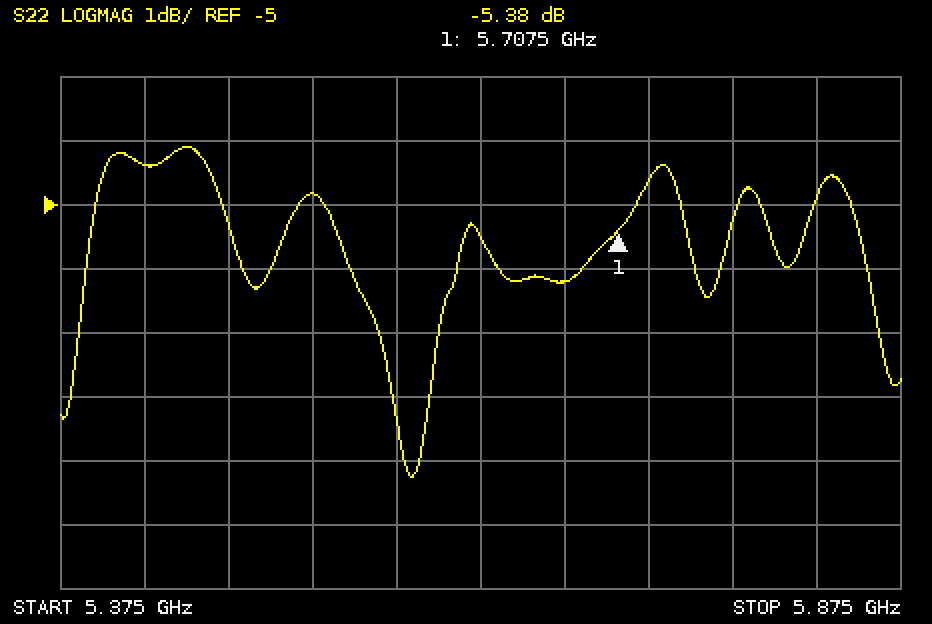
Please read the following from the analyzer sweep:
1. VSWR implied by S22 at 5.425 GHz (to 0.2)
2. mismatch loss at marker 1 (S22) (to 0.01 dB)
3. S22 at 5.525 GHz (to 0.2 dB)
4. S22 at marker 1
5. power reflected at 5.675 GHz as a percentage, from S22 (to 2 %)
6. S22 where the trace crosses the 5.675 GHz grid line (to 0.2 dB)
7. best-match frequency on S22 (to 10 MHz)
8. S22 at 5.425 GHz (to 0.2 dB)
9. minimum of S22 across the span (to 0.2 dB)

4.0
1.49 dB
-4.8 dB
-5.38 dB
24 %
-6.2 dB
5.58 GHz
-4.4 dB
-9.2 dB
